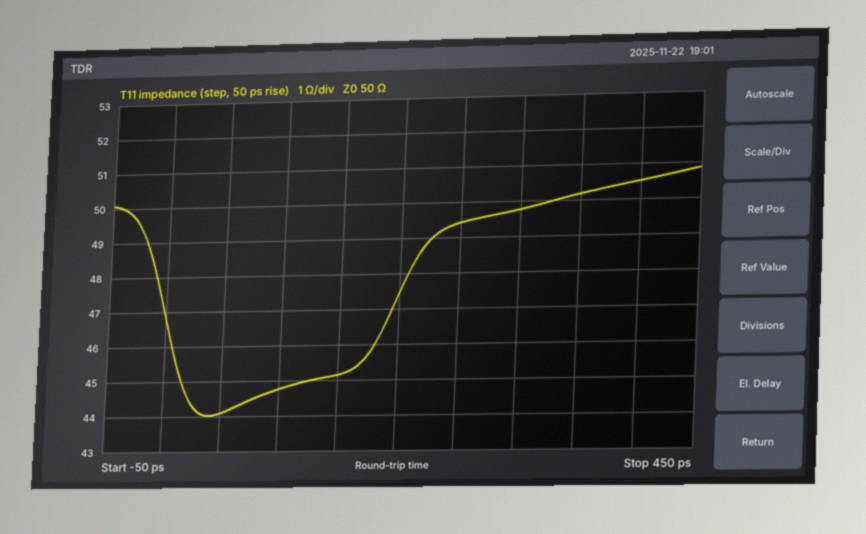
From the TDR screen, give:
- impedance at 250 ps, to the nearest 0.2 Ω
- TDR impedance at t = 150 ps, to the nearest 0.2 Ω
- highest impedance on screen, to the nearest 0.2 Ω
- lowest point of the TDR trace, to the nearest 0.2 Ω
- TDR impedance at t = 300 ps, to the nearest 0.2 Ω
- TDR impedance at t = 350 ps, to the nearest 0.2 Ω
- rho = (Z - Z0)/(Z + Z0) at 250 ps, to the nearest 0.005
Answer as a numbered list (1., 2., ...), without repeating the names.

1. 49.4 Ω
2. 45.2 Ω
3. 50.8 Ω
4. 44.0 Ω
5. 49.8 Ω
6. 50.2 Ω
7. -0.005
